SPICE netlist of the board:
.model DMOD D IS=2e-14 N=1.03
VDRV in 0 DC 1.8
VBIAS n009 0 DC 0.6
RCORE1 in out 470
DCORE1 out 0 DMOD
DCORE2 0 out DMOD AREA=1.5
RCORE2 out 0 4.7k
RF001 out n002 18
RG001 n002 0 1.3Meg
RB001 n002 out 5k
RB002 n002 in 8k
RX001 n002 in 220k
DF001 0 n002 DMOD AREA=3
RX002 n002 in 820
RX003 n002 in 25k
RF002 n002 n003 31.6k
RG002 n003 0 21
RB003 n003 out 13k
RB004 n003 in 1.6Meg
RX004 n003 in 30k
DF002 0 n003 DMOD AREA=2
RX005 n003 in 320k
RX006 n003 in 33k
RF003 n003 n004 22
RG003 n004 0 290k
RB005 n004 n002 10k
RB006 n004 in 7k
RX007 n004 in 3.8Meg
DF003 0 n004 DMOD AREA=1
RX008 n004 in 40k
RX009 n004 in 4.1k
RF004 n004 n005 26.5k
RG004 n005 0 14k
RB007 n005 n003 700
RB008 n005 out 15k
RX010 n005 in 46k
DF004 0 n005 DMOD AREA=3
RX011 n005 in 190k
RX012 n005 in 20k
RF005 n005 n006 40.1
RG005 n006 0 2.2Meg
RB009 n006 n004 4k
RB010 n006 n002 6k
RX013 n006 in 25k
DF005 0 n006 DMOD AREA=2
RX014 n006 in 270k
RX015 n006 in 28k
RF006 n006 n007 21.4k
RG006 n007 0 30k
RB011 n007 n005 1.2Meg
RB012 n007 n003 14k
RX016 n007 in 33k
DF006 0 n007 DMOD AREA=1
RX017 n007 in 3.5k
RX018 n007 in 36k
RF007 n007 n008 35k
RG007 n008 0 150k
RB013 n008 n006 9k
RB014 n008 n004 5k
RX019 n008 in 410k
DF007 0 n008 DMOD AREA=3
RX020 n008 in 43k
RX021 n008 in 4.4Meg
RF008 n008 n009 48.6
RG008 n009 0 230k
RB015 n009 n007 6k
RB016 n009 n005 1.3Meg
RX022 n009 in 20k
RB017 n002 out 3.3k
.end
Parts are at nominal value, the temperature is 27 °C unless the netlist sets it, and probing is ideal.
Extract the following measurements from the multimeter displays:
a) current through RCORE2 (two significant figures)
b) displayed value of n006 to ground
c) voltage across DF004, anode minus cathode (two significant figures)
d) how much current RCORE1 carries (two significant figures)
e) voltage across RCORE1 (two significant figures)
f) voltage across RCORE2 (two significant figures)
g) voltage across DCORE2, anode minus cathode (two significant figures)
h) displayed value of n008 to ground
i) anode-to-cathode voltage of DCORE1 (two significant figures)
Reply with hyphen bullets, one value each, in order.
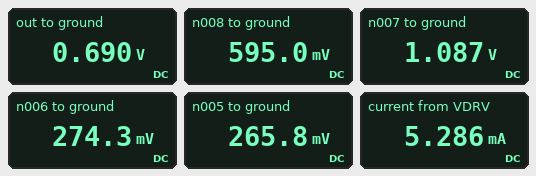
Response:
- 150 µA
- 274.3 mV
- -270 mV
- 2.4 mA
- 1.1 V
- 690 mV
- -690 mV
- 595.0 mV
- 690 mV
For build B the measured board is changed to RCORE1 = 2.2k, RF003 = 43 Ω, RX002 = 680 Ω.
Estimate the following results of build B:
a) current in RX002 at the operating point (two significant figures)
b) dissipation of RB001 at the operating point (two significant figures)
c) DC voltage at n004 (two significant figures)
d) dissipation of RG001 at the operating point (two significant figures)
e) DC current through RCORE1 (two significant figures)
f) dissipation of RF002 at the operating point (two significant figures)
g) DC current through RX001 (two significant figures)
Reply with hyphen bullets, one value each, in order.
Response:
- 1.6 mA
- 170 nW
- 73 mV
- 380 nW
- 510 µA
- 14 µW
- 5.0 µA
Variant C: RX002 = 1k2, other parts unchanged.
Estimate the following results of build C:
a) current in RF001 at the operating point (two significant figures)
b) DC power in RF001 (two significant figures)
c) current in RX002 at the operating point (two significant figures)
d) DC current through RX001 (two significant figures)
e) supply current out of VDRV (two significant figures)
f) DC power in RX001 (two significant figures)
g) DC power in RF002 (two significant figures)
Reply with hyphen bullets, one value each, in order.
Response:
- 930 µA
- 16 µW
- 910 µA
- 5.0 µA
- 4.9 mA
- 5.5 µW
- 14 µW
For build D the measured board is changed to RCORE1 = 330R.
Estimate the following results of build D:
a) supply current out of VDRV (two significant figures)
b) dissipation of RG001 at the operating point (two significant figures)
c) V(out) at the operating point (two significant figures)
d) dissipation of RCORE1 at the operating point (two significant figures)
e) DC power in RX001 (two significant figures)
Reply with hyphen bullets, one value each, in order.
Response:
- 6.3 mA
- 400 nW
- 700 mV
- 3.7 mW
- 5.3 µW
